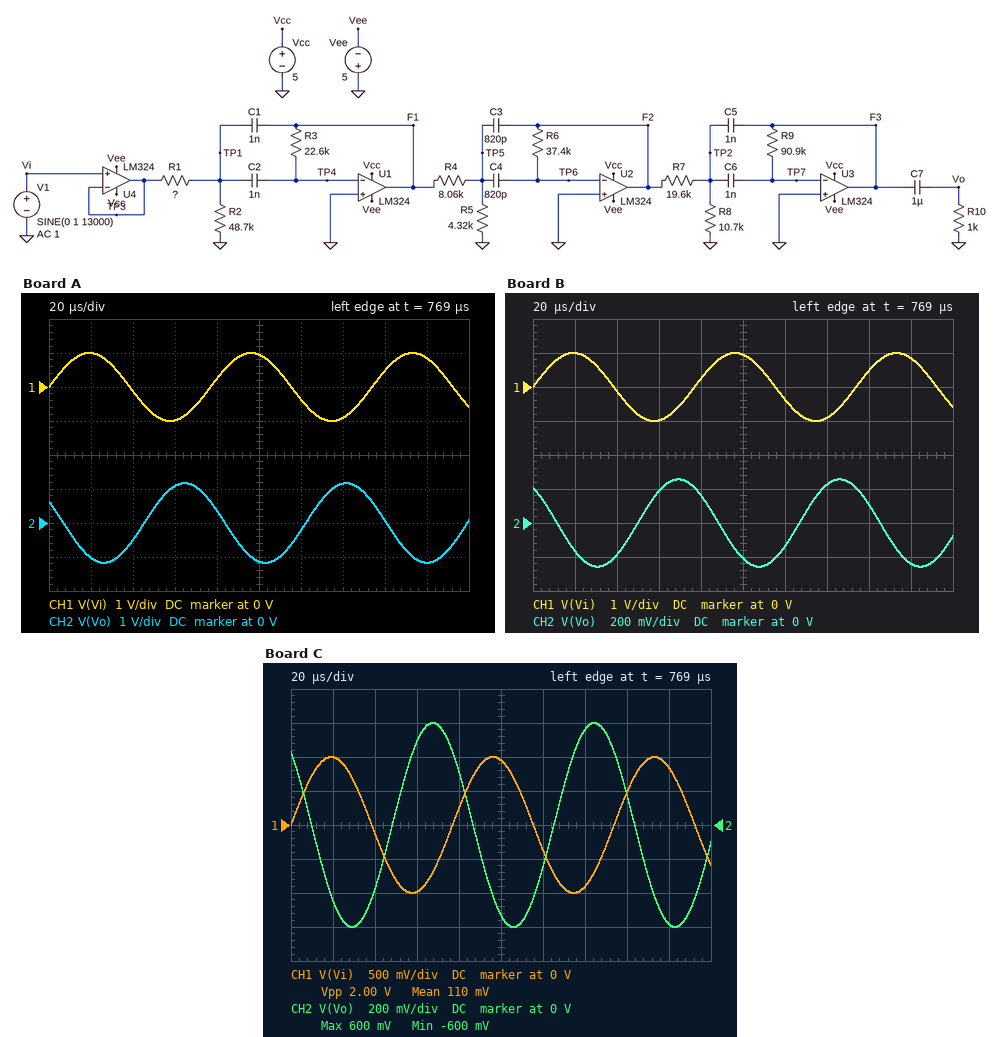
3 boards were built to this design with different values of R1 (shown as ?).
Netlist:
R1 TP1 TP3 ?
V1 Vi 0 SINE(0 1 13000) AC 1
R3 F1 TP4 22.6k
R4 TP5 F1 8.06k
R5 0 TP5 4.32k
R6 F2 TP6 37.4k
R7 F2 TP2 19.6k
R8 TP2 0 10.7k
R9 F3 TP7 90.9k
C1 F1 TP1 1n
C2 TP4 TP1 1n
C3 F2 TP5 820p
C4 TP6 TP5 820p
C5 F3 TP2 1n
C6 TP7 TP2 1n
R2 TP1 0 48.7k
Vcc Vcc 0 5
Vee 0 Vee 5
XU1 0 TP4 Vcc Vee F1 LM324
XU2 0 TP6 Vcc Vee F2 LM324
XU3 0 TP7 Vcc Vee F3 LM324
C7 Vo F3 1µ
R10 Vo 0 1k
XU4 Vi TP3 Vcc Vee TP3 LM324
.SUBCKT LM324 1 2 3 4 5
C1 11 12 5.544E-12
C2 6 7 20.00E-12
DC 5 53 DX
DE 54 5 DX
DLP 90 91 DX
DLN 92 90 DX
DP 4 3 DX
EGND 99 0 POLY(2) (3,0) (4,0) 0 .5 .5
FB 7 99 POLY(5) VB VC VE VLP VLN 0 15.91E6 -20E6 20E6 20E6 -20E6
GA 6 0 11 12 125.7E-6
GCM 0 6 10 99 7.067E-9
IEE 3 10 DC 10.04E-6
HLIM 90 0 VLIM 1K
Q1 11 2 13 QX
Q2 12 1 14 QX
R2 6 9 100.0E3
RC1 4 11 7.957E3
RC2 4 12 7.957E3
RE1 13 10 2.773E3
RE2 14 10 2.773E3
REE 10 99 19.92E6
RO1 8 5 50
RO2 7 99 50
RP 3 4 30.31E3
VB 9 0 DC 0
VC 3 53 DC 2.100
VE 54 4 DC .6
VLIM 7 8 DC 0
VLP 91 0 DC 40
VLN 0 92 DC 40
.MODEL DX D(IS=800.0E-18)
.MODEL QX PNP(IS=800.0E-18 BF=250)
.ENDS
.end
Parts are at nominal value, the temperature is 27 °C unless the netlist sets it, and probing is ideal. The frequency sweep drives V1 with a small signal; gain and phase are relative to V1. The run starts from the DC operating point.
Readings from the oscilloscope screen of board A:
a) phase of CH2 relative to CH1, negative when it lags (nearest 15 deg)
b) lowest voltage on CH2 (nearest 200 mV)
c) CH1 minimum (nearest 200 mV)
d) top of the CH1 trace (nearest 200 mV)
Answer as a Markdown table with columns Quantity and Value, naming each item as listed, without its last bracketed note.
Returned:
| Quantity | Value |
|---|---|
| phase of CH2 relative to CH1, negative when it lags | 150 deg |
| lowest voltage on CH2 | -1.2 V |
| CH1 minimum | -1.0 V |
| top of the CH1 trace | 1.0 V |
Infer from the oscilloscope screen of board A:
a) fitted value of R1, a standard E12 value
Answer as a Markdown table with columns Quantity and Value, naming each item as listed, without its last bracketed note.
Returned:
| Quantity | Value |
|---|---|
| fitted value of R1, a standard E12 value | 10 kΩ |
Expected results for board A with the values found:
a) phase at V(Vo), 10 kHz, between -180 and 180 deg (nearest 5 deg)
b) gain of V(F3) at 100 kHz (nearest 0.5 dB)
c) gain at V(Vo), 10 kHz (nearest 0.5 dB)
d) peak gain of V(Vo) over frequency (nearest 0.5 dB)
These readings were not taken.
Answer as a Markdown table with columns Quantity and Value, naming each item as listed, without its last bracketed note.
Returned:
| Quantity | Value |
|---|---|
| phase at V(Vo), 10 kHz, between -180 and 180 deg | -160 deg |
| gain of V(F3) at 100 kHz | -50.5 dB |
| gain at V(Vo), 10 kHz | 1.0 dB |
| peak gain of V(Vo) over frequency | 1.5 dB |
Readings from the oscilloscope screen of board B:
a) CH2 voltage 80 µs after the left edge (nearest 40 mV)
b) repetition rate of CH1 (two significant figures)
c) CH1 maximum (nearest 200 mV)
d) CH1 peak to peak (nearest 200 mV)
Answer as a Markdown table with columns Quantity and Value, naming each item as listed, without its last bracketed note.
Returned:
| Quantity | Value |
|---|---|
| CH2 voltage 80 µs after the left edge | 160 mV |
| repetition rate of CH1 | 13 kHz |
| CH1 maximum | 1.0 V |
| CH1 peak to peak | 2.0 V |
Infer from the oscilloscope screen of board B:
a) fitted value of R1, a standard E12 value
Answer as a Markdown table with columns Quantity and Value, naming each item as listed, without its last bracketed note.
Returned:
| Quantity | Value |
|---|---|
| fitted value of R1, a standard E12 value | 39 kΩ |
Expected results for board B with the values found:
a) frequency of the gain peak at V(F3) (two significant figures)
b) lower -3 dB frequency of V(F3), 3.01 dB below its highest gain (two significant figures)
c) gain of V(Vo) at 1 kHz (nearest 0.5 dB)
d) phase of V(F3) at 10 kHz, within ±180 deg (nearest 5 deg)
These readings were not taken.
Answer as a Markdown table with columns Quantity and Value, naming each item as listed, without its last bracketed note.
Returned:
| Quantity | Value |
|---|---|
| frequency of the gain peak at V(F3) | 7.0 kHz |
| lower -3 dB frequency of V(F3), 3.01 dB below its highest gain | 5.5 kHz |
| gain of V(Vo) at 1 kHz | -59.5 dB |
| phase of V(F3) at 10 kHz, within ±180 deg | 165 deg |
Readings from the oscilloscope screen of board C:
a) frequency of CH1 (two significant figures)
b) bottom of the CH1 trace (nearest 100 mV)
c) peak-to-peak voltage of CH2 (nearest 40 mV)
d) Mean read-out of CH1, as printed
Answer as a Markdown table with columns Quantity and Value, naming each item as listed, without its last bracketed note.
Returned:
| Quantity | Value |
|---|---|
| frequency of CH1 | 13 kHz |
| bottom of the CH1 trace | -1.0 V |
| peak-to-peak voltage of CH2 | 1.20 V |
| Mean read-out of CH1, as printed | 110 mV |
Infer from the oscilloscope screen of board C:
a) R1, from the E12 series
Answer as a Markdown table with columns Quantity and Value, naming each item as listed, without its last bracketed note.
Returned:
| Quantity | Value |
|---|---|
| R1, from the E12 series | 18 kΩ |
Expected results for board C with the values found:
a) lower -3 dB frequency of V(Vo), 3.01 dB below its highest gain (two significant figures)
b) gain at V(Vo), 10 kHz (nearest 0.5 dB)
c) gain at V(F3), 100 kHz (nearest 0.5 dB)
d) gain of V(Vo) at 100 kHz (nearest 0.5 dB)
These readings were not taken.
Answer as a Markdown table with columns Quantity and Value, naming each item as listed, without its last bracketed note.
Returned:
| Quantity | Value |
|---|---|
| lower -3 dB frequency of V(Vo), 3.01 dB below its highest gain | 5.7 kHz |
| gain at V(Vo), 10 kHz | -4.0 dB |
| gain at V(F3), 100 kHz | -56.0 dB |
| gain of V(Vo) at 100 kHz | -56.0 dB |
